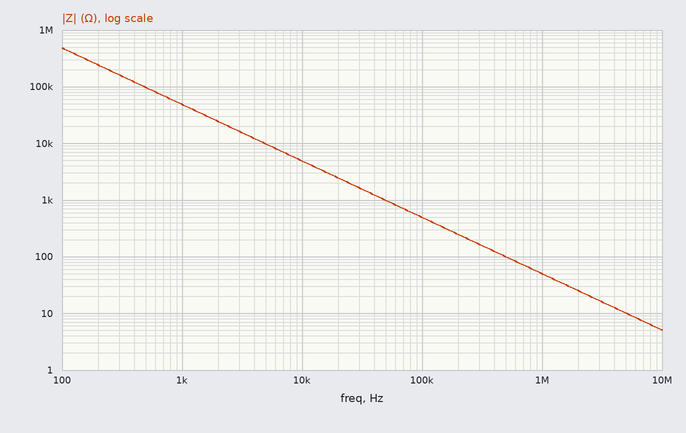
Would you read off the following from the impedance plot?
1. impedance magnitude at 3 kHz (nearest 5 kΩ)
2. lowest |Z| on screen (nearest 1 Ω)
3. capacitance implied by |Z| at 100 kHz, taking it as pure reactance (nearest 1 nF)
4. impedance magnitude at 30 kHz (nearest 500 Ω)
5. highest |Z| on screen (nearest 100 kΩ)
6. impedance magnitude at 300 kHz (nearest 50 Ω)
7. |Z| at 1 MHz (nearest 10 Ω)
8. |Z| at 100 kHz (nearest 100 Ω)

15 kΩ
5 Ω
3 nF
1.5 kΩ
500 kΩ
150 Ω
50 Ω
500 Ω
